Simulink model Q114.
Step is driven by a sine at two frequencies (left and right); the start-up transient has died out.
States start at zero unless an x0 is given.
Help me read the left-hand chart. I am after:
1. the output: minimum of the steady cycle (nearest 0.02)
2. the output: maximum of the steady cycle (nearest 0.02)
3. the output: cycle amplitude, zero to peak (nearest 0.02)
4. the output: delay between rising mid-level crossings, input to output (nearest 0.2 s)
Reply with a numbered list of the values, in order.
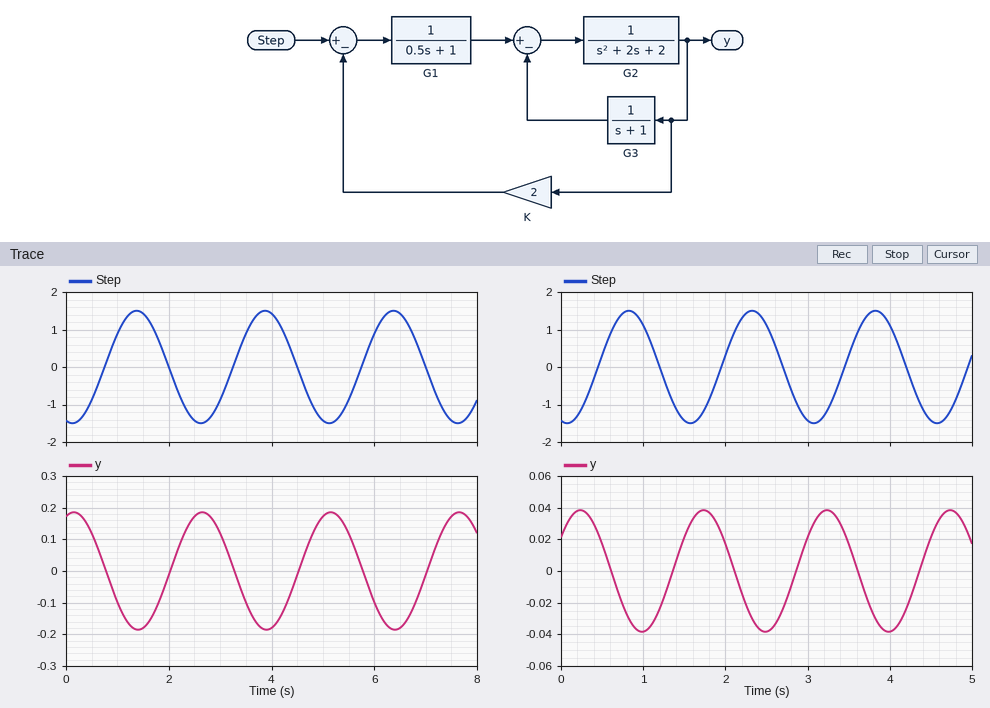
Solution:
1. -0.18
2. 0.18
3. 0.18
4. 1.2 s
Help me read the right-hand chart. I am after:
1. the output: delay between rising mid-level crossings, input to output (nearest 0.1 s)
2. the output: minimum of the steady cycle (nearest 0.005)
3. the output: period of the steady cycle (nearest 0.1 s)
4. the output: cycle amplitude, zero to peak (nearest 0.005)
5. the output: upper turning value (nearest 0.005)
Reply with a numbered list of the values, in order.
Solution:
1. 0.9 s
2. -0.040
3. 1.5 s
4. 0.040
5. 0.040
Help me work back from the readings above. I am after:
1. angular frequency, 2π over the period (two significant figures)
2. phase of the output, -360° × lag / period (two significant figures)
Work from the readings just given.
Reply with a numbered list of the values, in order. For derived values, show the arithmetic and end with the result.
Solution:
1. 2π / 1.5 = 4.2 rad/s
2. -360 × 0.9 / 1.5 = -220°
